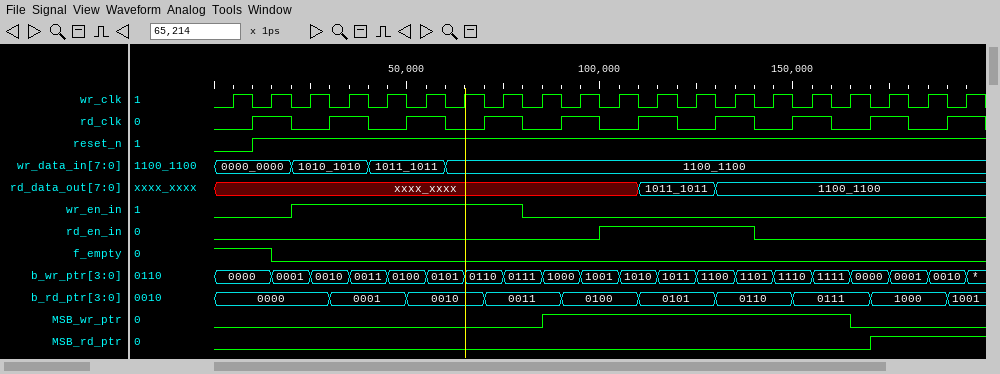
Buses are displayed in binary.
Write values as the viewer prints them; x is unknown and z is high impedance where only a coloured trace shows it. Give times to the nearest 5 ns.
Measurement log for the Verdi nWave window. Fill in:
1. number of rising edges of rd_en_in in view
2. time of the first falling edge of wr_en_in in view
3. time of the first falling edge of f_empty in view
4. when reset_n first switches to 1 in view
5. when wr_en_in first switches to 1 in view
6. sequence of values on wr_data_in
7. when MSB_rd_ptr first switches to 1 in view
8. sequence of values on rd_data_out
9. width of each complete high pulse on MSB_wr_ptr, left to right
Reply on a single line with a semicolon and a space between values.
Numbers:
1; 80 ns; 15 ns; 10 ns; 20 ns; 0000_0000, 1010_1010, 1011_1011, 1100_1100; 170 ns; xxxx_xxxx, 1011_1011, 1100_1100; 80 ns
